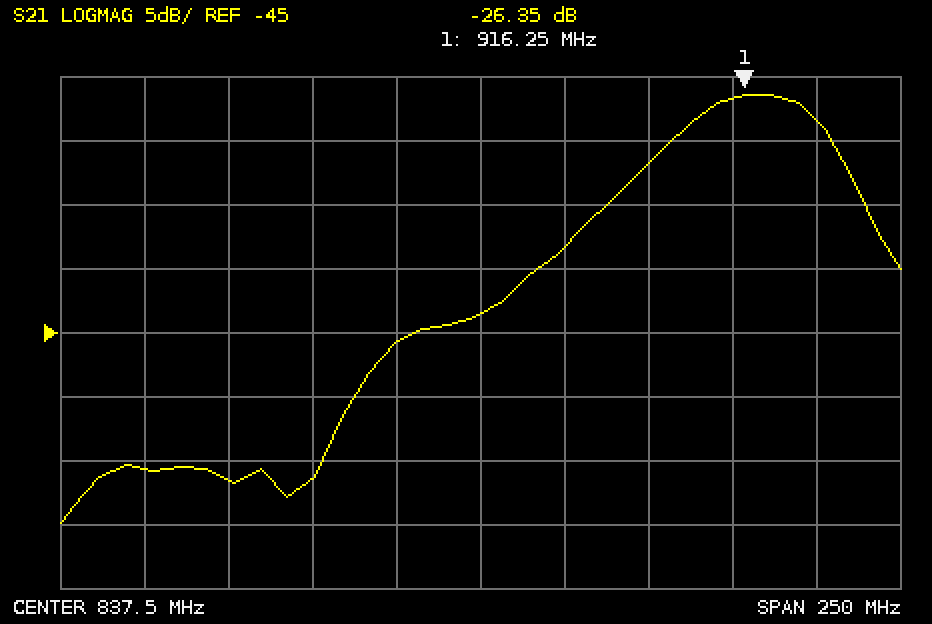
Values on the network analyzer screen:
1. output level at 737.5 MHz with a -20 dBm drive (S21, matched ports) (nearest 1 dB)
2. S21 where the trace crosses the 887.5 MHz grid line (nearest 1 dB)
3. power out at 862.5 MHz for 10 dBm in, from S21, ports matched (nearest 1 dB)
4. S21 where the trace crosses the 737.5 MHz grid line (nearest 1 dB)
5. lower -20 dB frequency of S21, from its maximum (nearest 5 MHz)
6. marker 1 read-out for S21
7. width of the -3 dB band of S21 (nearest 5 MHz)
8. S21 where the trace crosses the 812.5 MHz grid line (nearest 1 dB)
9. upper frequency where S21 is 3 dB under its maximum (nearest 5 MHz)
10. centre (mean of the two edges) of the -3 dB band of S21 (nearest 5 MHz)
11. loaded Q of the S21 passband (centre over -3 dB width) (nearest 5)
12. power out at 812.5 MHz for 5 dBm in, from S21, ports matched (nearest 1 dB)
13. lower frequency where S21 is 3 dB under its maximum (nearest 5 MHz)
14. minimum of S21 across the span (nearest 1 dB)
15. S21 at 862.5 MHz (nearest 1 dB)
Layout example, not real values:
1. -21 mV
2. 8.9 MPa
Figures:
1. -76 dBm
2. -32 dB
3. -28 dBm
4. -56 dB
5. 810 MHz
6. -26.35 dB
7. 45 MHz
8. -46 dB
9. 940 MHz
10. 920 MHz
11. 20
12. -41 dBm
13. 895 MHz
14. -60 dB
15. -38 dB
